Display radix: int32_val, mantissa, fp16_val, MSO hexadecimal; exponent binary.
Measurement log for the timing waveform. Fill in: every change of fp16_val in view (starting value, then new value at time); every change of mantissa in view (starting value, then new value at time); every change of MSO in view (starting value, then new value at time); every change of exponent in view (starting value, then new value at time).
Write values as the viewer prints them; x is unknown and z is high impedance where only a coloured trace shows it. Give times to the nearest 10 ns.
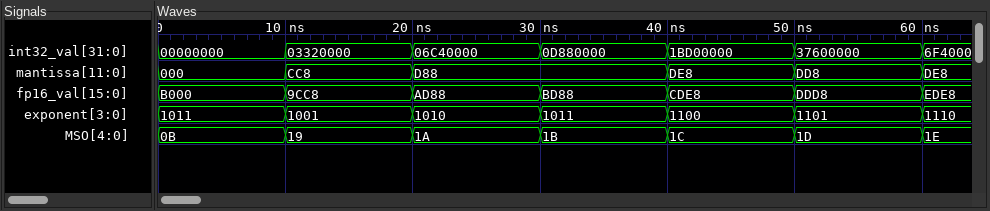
B000, 9CC8 at 10 ns, AD88 at 20 ns, BD88 at 30 ns, CDE8 at 40 ns, DDD8 at 50 ns, EDE8 at 60 ns
000, CC8 at 10 ns, D88 at 20 ns, DE8 at 40 ns, DD8 at 50 ns, DE8 at 60 ns
0B, 19 at 10 ns, 1A at 20 ns, 1B at 30 ns, 1C at 40 ns, 1D at 50 ns, 1E at 60 ns
1011, 1001 at 10 ns, 1010 at 20 ns, 1011 at 30 ns, 1100 at 40 ns, 1101 at 50 ns, 1110 at 60 ns
